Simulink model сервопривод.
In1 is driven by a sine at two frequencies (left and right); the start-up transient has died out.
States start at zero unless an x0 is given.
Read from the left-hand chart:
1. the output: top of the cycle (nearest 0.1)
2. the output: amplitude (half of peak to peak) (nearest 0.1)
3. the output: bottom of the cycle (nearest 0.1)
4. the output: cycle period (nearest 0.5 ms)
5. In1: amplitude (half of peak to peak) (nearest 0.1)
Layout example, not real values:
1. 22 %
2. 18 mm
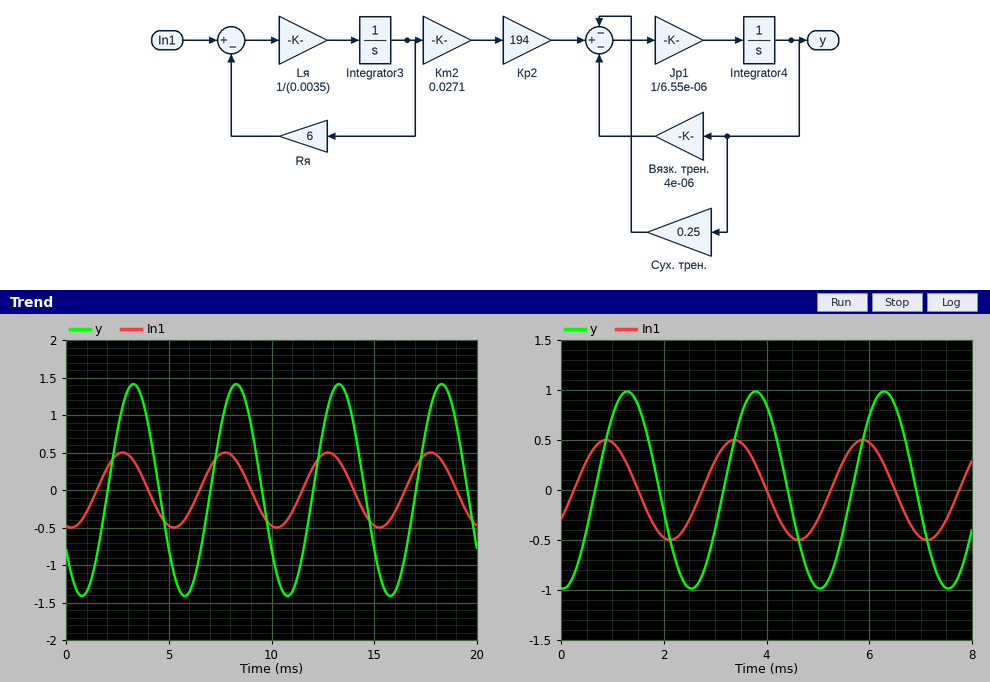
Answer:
1. 1.4
2. 1.4
3. -1.4
4. 5.0 ms
5. 0.5
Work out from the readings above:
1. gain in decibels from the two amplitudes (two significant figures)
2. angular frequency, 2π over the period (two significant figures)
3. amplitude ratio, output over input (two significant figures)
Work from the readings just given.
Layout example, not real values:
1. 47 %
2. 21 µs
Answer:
1. 8.9 dB
2. 1.3 rad/ms
3. 2.8
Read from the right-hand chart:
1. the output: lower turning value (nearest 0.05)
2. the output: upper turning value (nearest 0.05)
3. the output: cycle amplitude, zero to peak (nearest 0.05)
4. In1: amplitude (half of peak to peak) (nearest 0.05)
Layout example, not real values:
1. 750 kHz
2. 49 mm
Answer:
1. -1.00
2. 1.00
3. 1.00
4. 0.50
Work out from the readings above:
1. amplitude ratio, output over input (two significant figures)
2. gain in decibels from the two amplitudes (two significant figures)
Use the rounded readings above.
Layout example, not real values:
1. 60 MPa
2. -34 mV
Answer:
1. 2.0
2. 6.0 dB
